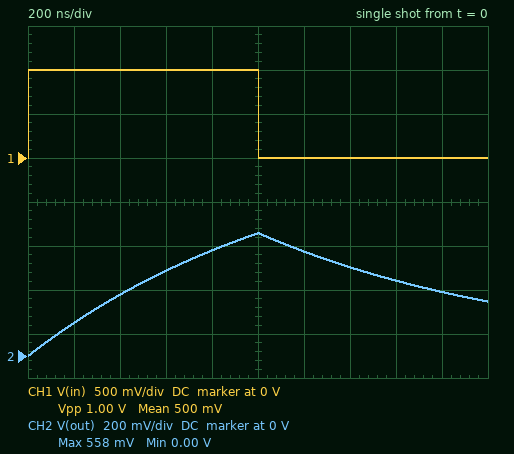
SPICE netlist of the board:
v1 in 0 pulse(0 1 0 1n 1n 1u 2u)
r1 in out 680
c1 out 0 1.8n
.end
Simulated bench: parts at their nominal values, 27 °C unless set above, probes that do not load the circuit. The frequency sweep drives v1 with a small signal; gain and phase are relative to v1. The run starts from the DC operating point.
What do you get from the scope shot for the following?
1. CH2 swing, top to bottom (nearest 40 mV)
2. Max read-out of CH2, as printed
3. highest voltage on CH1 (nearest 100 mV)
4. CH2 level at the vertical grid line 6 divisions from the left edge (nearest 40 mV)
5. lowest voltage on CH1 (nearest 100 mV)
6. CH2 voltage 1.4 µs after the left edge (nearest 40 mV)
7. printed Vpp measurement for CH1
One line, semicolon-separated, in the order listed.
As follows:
560 mV; 558 mV; 1.0 V; 480 mV; 0 V; 400 mV; 1.00 V
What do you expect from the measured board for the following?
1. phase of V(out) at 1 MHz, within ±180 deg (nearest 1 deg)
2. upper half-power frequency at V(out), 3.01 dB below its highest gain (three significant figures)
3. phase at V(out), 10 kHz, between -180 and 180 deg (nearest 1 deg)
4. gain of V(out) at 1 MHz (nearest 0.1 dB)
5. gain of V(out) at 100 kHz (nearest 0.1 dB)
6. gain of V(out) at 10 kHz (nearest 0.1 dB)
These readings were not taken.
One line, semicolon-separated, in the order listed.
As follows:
-83 deg; 130 kHz; -4 deg; -17.8 dB; -2.0 dB; 0 dB
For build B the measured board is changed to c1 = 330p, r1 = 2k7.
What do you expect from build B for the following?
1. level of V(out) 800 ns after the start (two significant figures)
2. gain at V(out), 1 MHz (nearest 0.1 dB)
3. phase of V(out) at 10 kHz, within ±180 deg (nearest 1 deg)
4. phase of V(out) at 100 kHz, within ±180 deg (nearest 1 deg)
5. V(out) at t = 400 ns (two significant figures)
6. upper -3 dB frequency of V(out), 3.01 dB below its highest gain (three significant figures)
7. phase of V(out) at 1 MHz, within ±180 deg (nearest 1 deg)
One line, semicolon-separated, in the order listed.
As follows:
590 mV; -15.1 dB; -3 deg; -29 deg; 360 mV; 179 kHz; -80 deg
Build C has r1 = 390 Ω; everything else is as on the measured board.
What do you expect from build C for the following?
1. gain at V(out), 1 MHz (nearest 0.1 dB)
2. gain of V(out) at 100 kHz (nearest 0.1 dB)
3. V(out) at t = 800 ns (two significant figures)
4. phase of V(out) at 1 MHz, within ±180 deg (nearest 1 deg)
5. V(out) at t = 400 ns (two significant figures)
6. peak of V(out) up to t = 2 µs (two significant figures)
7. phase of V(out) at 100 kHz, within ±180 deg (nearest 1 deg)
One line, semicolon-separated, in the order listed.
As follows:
-13.1 dB; -0.8 dB; 680 mV; -77 deg; 430 mV; 760 mV; -24 deg
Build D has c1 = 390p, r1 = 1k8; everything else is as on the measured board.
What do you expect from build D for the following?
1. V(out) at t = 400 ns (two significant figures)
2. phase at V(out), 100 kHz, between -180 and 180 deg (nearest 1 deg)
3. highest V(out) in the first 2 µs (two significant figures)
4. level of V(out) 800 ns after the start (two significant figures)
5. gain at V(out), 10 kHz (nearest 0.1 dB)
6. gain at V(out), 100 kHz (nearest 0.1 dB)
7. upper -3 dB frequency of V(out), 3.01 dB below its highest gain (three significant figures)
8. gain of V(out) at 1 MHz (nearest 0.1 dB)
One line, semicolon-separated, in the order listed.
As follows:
430 mV; -24 deg; 760 mV; 680 mV; 0 dB; -0.8 dB; 227 kHz; -13.1 dB
